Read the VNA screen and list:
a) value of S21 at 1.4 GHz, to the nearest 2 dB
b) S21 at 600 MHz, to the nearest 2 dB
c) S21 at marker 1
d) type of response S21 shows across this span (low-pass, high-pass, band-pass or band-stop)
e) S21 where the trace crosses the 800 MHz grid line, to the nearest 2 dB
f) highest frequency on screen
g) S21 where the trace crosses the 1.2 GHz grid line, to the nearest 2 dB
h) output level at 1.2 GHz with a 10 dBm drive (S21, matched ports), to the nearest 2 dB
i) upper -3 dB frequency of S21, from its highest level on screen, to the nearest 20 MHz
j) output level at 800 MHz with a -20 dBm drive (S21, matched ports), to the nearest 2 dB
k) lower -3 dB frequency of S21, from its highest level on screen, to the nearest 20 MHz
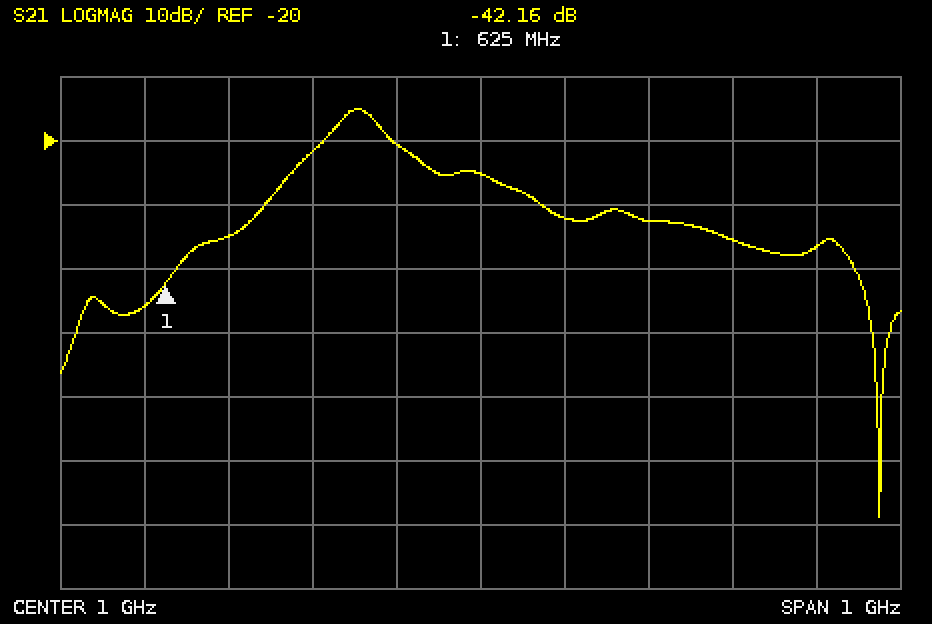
-36 dB
-46 dB
-42.16 dB
band-pass
-22 dB
1.5 GHz
-32 dB
-22 dBm
880 MHz
-42 dBm
820 MHz
